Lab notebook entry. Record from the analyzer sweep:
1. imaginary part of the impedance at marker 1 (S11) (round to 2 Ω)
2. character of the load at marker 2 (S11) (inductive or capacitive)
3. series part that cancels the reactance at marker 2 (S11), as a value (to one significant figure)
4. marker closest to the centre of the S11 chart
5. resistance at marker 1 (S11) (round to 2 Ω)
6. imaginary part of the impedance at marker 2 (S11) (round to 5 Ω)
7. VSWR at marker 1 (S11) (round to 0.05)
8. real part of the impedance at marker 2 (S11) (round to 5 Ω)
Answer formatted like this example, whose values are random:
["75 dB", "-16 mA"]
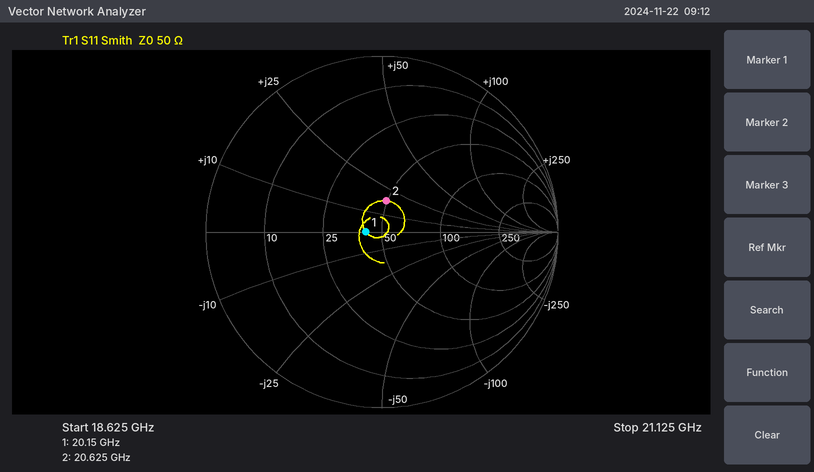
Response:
["0 Ω", "inductive", "400 fF", "marker 1", "42 Ω", "+20 Ω", "1.20", "50 Ω"]
